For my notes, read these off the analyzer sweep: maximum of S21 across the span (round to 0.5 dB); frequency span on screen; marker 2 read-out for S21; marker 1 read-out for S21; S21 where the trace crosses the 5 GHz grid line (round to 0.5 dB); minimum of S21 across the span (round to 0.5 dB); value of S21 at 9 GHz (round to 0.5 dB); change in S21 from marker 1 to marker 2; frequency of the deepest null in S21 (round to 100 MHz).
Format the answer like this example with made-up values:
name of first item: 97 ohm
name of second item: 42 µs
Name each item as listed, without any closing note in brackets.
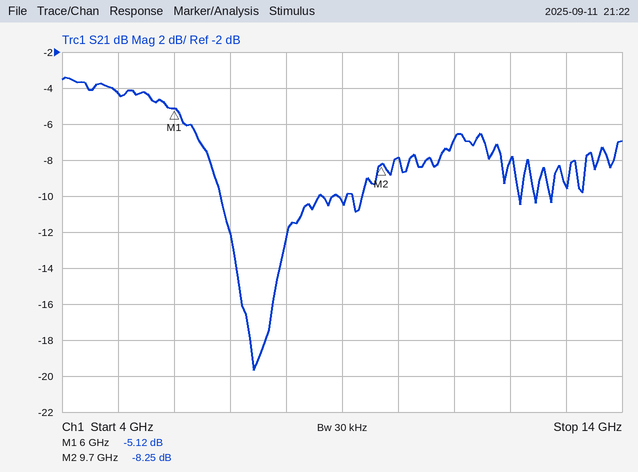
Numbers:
maximum of S21 across the span: -3.5 dB
frequency span on screen: 10 GHz
marker 2 read-out for S21: -8.25 dB
marker 1 read-out for S21: -5.12 dB
S21 where the trace crosses the 5 GHz grid line: -4.5 dB
minimum of S21 across the span: -19.5 dB
value of S21 at 9 GHz: -10.5 dB
change in S21 from marker 1 to marker 2: -3.13 dB
frequency of the deepest null in S21: 7.4 GHz
